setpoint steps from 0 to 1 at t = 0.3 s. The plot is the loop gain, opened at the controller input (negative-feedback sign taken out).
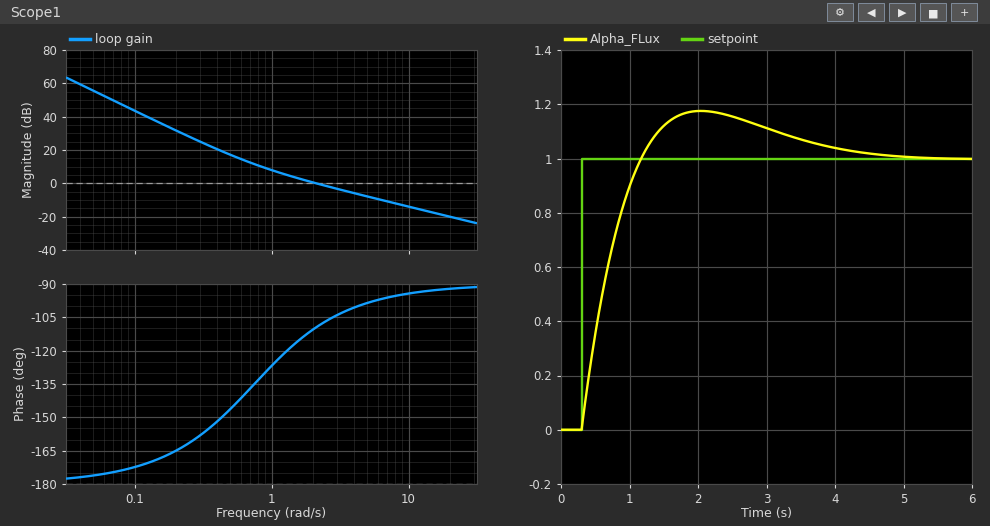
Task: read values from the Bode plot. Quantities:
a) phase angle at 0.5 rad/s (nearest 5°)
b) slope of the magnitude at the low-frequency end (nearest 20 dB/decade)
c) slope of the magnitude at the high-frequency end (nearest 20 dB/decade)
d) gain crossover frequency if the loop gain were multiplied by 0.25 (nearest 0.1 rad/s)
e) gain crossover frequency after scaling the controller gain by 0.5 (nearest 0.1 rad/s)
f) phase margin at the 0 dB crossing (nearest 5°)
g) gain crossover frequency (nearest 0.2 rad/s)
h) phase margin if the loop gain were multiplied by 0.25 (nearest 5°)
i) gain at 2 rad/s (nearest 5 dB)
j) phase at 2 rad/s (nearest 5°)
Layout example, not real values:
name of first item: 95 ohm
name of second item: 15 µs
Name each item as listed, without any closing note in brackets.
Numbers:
phase angle at 0.5 rad/s: -145°
slope of the magnitude at the low-frequency end: -40 dB/decade
slope of the magnitude at the high-frequency end: -20 dB/decade
gain crossover frequency if the loop gain were multiplied by 0.25: 0.7 rad/s
gain crossover frequency after scaling the controller gain by 0.5: 1.2 rad/s
phase margin at the 0 dB crossing: 70°
gain crossover frequency: 2.2 rad/s
phase margin if the loop gain were multiplied by 0.25: 45°
gain at 2 rad/s: 0 dB
phase at 2 rad/s: -110°
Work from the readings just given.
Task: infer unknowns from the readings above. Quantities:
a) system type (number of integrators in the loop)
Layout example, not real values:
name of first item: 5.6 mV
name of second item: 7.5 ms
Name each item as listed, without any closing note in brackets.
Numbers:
system type: 2
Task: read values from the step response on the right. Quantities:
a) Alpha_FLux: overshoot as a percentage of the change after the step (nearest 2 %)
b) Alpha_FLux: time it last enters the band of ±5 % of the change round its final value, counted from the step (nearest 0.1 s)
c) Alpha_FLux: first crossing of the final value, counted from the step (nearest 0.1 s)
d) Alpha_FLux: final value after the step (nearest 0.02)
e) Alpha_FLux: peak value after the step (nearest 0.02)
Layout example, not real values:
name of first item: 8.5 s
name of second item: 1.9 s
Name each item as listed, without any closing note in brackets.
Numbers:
Alpha_FLux: overshoot as a percentage of the change after the step: 18 %
Alpha_FLux: time it last enters the band of ±5 % of the change round its final value, counted from the step: 3.5 s
Alpha_FLux: first crossing of the final value, counted from the step: 0.9 s
Alpha_FLux: final value after the step: 1.00
Alpha_FLux: peak value after the step: 1.18
